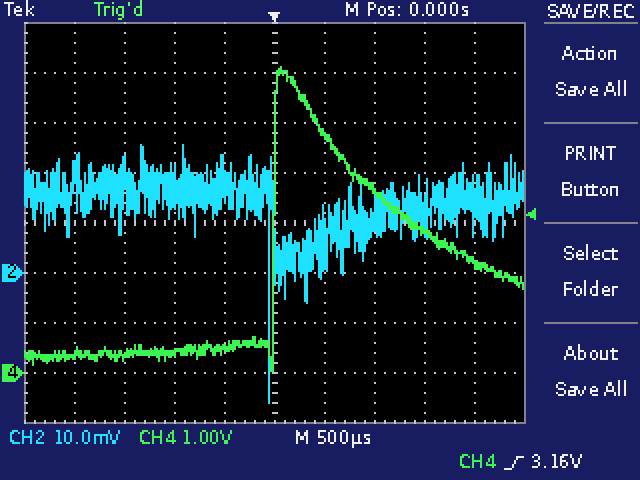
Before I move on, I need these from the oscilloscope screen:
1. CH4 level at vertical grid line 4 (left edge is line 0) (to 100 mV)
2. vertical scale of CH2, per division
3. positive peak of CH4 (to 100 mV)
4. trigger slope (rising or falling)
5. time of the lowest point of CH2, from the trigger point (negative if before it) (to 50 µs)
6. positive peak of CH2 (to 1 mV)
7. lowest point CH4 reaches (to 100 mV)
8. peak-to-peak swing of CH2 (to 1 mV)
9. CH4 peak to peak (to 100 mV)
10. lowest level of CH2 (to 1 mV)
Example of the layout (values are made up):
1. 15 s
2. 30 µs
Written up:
1. 500 mV
2. 10 mV
3. 6.1 V
4. rising
5. -50 µs
6. 26 mV
7. 0.0 V
8. 52 mV
9. 6.1 V
10. -26 mV
